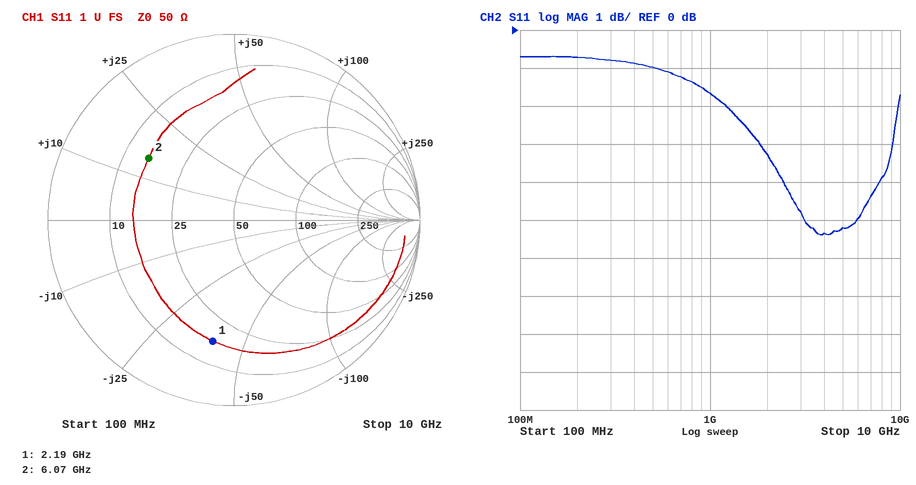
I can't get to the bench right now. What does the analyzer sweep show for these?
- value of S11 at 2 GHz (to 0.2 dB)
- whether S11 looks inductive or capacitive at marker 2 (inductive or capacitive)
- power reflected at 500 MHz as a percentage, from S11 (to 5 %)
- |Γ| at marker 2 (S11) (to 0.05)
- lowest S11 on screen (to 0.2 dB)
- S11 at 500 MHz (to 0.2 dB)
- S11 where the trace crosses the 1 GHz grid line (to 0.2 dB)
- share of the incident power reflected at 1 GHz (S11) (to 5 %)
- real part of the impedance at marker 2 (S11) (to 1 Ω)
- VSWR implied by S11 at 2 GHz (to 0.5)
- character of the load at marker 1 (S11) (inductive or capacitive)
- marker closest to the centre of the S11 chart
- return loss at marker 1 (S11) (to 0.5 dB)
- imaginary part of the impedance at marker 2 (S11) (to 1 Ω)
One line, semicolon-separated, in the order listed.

-3.2 dB; inductive; 80 %; 0.55; -5.4 dB; -1.0 dB; -1.6 dB; 70 %; 15 Ω; 5.5; capacitive; marker 2; 3.5 dB; +15 Ω
